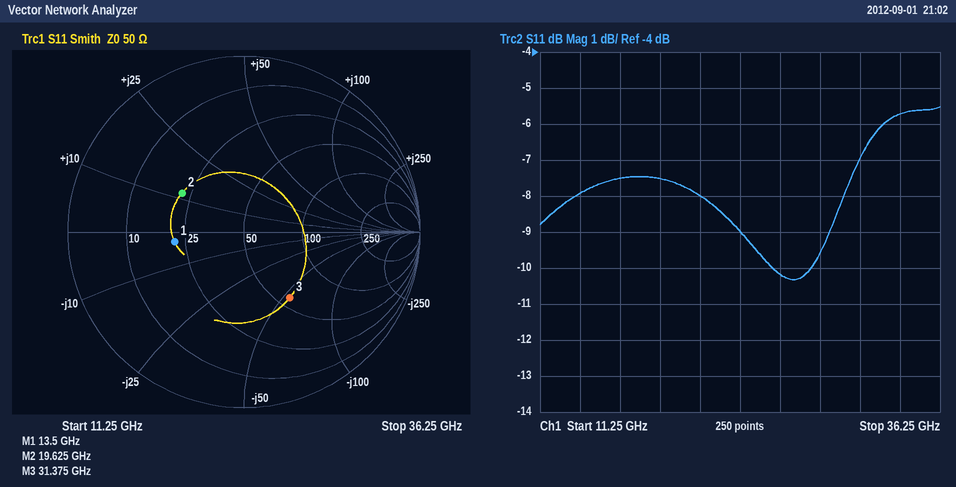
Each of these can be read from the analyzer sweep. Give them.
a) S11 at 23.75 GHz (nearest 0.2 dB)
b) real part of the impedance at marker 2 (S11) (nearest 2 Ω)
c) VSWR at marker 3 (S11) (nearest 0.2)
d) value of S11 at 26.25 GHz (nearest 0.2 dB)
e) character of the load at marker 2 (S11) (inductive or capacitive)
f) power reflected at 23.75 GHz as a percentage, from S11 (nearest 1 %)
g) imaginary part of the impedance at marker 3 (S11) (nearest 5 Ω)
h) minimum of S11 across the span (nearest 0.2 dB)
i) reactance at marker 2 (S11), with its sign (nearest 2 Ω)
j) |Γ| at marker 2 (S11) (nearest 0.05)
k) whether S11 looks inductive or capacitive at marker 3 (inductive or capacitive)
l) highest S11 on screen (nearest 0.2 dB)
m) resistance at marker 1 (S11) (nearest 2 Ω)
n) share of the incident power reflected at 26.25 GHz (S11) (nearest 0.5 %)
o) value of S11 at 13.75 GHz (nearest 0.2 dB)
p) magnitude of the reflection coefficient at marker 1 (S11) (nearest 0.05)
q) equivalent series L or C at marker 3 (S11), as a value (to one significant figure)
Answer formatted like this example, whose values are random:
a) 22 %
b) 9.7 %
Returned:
a) -9.0 dB
b) 22 Ω
c) 2.6
d) -10.2 dB
e) inductive
f) 13 %
g) -55 Ω
h) -10.4 dB
i) +12 Ω
j) 0.40
k) capacitive
l) -5.6 dB
m) 22 Ω
n) 9.5 %
o) -8.0 dB
p) 0.40
q) 90 fF
